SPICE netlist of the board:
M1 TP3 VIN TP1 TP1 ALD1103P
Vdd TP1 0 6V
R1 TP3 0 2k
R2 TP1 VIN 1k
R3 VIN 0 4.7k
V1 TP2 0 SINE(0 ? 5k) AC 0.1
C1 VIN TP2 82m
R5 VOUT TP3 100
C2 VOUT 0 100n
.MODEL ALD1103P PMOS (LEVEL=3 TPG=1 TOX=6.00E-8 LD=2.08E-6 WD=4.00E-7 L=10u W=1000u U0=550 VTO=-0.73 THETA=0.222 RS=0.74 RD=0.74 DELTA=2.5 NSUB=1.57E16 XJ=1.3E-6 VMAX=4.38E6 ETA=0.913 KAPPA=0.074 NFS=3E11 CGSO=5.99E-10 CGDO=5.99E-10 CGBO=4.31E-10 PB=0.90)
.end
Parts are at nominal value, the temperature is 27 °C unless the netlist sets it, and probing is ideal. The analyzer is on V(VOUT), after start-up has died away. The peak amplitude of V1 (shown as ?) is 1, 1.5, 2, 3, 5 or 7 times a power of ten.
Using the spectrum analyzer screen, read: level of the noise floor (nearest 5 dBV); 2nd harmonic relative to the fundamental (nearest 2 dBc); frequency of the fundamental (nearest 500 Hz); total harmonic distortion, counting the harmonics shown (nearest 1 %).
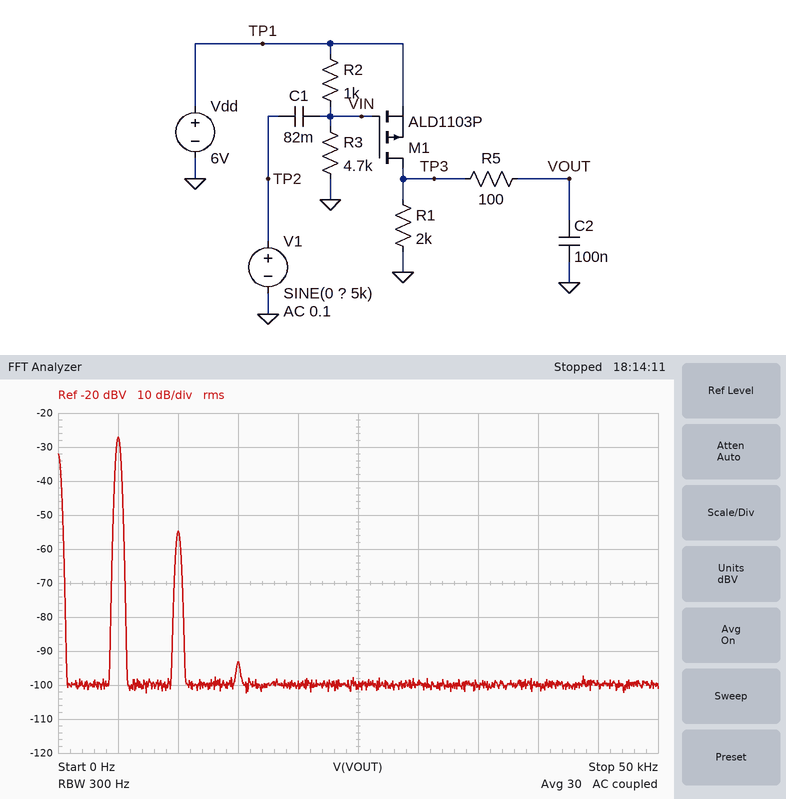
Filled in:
-100 dBV
-28 dBc
5.0 kHz
4 %
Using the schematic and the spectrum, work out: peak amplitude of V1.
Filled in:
150 mV
